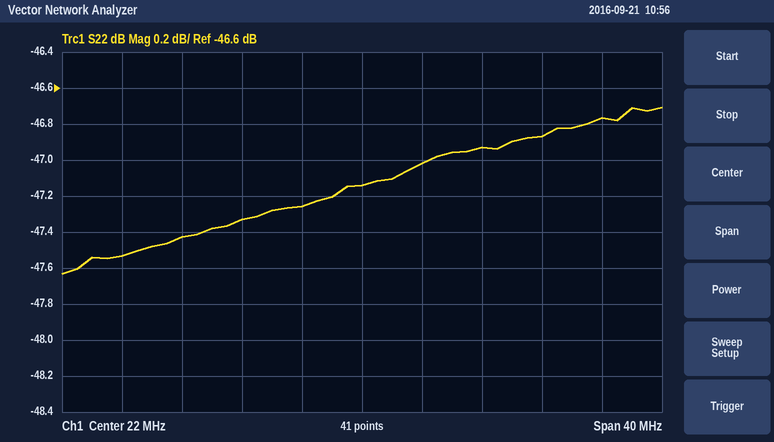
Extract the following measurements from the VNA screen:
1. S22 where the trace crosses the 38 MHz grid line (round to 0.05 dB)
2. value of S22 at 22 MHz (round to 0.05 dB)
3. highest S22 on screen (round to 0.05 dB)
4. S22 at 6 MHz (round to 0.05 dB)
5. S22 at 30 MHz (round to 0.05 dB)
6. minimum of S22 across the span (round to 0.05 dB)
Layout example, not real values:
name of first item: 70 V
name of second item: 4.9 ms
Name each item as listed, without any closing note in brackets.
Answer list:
S22 where the trace crosses the 38 MHz grid line: -46.75 dB
value of S22 at 22 MHz: -47.15 dB
highest S22 on screen: -46.70 dB
S22 at 6 MHz: -47.55 dB
S22 at 30 MHz: -46.95 dB
minimum of S22 across the span: -47.65 dB
